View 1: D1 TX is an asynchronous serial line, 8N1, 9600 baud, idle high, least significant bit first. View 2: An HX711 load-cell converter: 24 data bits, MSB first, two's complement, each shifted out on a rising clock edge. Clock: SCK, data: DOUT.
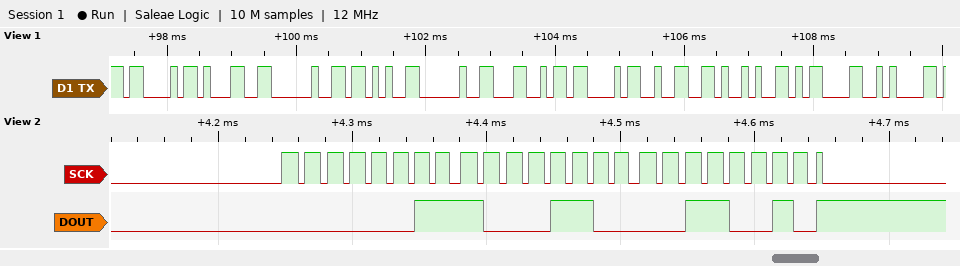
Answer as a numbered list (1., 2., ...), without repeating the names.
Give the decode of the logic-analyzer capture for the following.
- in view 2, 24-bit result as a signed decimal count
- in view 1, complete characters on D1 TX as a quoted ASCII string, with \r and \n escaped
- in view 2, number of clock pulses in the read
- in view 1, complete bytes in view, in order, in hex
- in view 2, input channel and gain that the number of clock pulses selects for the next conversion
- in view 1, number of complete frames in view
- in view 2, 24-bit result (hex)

1. 232498
2. "C1 + LC2)\r\n"
3. 25
4. 0x43 0x31 0x20 0x2B 0x20 0x4C 0x43 0x32 0x29 0x0D 0x0A
5. channel A, gain 128
6. 11
7. 0x038C32
